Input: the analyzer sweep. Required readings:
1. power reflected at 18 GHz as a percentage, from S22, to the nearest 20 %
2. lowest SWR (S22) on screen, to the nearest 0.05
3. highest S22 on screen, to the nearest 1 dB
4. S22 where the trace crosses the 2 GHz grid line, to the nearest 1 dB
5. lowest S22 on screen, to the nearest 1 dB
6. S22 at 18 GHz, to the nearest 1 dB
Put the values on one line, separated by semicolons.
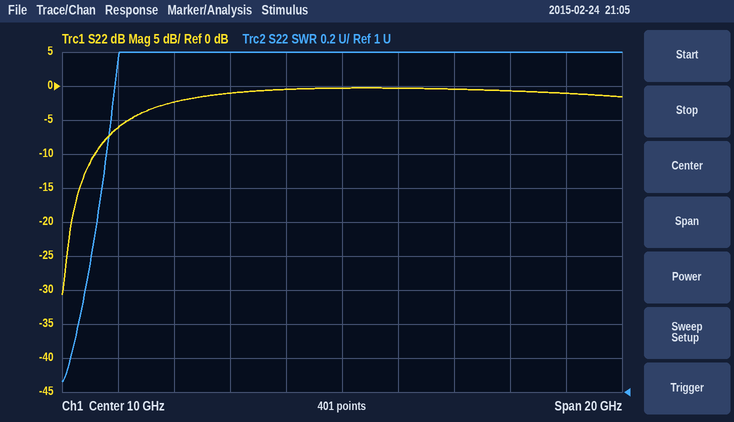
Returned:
80 %; 1.05; 0 dB; -6 dB; -31 dB; -1 dB
